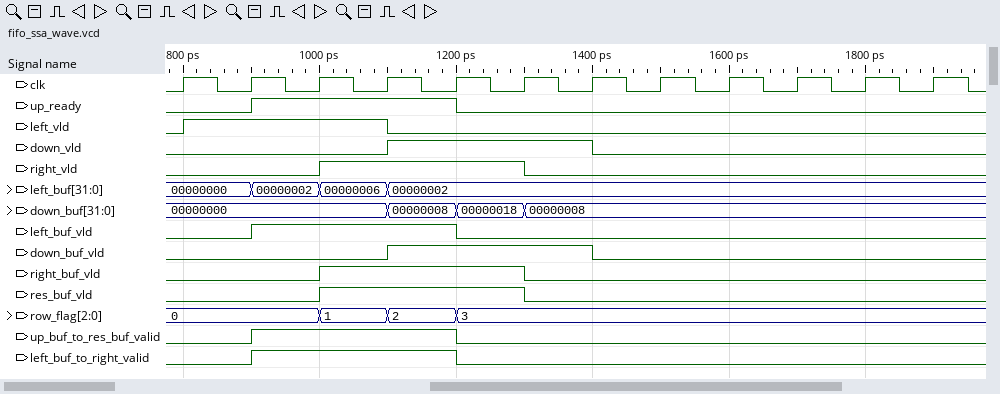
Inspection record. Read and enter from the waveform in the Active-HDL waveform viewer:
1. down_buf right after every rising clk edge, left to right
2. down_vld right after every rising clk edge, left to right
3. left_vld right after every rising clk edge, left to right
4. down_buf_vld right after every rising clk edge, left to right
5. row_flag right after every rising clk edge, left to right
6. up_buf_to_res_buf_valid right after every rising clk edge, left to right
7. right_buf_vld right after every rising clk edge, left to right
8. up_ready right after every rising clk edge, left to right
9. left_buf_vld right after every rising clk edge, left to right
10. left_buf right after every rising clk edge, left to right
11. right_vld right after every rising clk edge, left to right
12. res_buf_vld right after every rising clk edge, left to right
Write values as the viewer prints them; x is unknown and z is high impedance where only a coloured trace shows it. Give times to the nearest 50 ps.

00000000, 00000000, 00000000, 00000008, 00000018, 00000008, 00000008, 00000008, 00000008, 00000008, 00000008, 00000008
0 0 0 1 1 1 0 0 0 0 0 0
1 1 1 0 0 0 0 0 0 0 0 0
0 0 0 1 1 1 0 0 0 0 0 0
0, 0, 1, 2, 3, 3, 3, 3, 3, 3, 3, 3
0 1 1 1 0 0 0 0 0 0 0 0
0 0 1 1 1 0 0 0 0 0 0 0
0 1 1 1 0 0 0 0 0 0 0 0
0 1 1 1 0 0 0 0 0 0 0 0
00000000, 00000002, 00000006, 00000002, 00000002, 00000002, 00000002, 00000002, 00000002, 00000002, 00000002, 00000002
0 0 1 1 1 0 0 0 0 0 0 0
0 0 1 1 1 0 0 0 0 0 0 0
